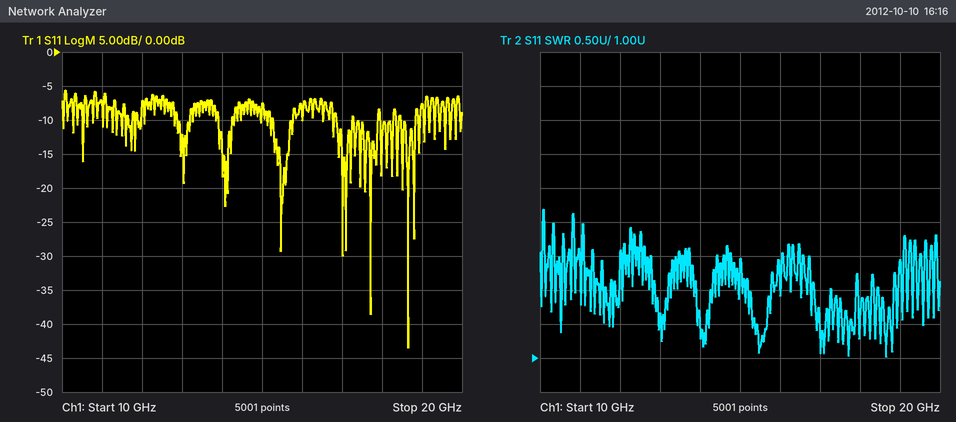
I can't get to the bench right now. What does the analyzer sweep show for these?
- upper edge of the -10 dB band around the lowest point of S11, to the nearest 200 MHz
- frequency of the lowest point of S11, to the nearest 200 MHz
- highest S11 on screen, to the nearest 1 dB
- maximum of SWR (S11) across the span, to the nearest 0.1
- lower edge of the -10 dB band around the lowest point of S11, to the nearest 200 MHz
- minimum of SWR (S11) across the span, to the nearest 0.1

18.8 GHz
18.6 GHz
-6 dB
3.2
18.4 GHz
1.0
